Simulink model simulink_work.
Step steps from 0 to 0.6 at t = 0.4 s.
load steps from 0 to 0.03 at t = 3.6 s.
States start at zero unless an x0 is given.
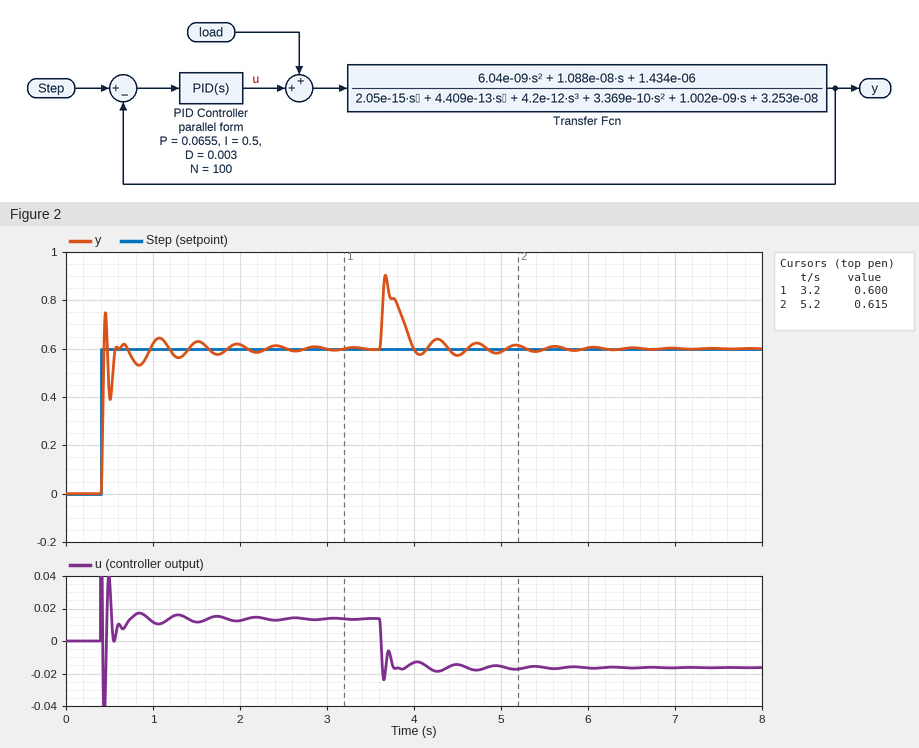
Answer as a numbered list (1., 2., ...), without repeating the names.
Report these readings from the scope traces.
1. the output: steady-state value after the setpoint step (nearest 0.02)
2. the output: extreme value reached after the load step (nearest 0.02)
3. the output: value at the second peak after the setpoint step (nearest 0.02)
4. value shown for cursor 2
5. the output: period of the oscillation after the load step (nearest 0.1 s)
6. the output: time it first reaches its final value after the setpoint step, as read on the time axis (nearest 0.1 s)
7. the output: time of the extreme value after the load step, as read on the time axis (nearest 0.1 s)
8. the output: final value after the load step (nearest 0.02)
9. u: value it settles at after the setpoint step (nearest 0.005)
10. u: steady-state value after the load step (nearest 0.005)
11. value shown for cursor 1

1. 0.60
2. 0.90
3. 0.62
4. 0.615
5. 0.6 s
6. 0.4 s
7. 3.7 s
8. 0.60
9. 0.015
10. -0.015
11. 0.600
